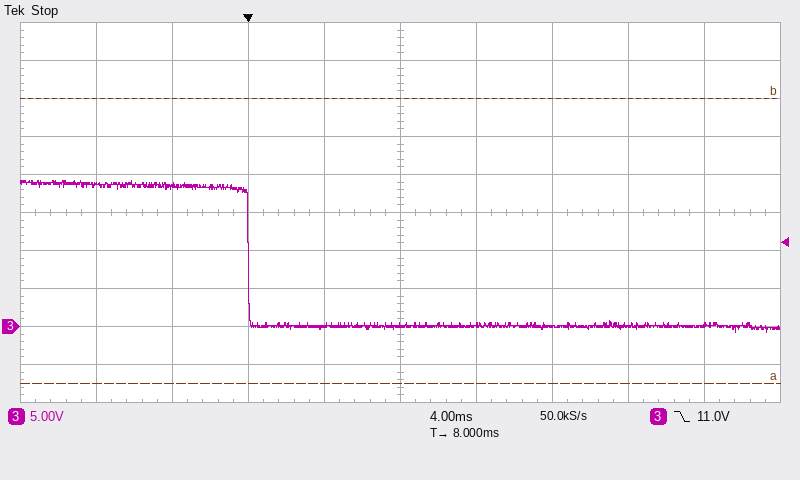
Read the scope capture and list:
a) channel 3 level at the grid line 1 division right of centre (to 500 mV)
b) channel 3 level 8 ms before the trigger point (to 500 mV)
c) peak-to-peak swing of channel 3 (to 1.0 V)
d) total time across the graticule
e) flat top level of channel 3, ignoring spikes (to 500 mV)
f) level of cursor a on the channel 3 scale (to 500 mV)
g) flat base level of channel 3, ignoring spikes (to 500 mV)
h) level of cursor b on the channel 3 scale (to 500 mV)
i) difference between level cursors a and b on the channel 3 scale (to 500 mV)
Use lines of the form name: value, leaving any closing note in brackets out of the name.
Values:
channel 3 level at the grid line 1 division right of centre: 0.0 V
channel 3 level 8 ms before the trigger point: 18.5 V
peak-to-peak swing of channel 3: 20.0 V
total time across the graticule: 40 ms
flat top level of channel 3, ignoring spikes: 18.5 V
level of cursor a on the channel 3 scale: -7.5 V
flat base level of channel 3, ignoring spikes: 0.0 V
level of cursor b on the channel 3 scale: 30.0 V
difference between level cursors a and b on the channel 3 scale: 37.5 V
